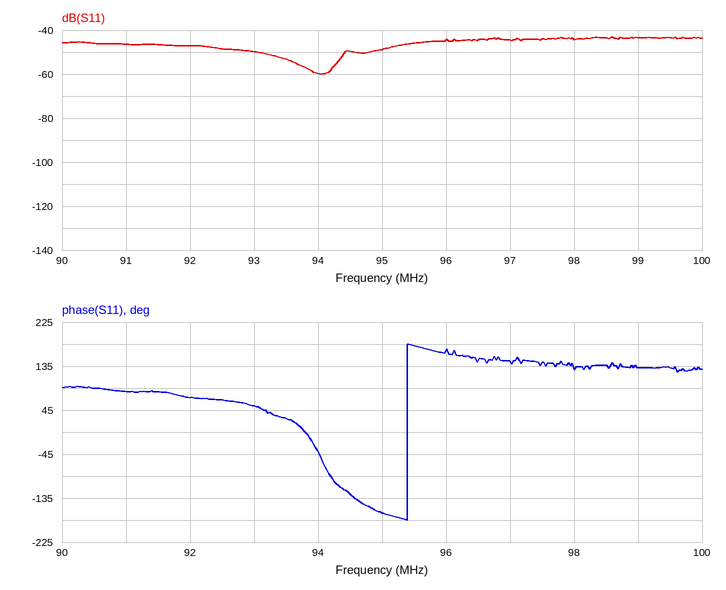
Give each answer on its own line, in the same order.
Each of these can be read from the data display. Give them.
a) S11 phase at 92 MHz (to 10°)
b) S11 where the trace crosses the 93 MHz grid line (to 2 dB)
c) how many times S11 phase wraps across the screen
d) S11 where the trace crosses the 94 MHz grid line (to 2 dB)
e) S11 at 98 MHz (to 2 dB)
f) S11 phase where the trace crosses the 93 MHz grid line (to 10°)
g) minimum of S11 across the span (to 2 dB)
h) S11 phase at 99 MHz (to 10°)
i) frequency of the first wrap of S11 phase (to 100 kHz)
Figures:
70°
-50 dB
1
-60 dB
-44 dB
50°
-60 dB
130°
95.4 MHz
